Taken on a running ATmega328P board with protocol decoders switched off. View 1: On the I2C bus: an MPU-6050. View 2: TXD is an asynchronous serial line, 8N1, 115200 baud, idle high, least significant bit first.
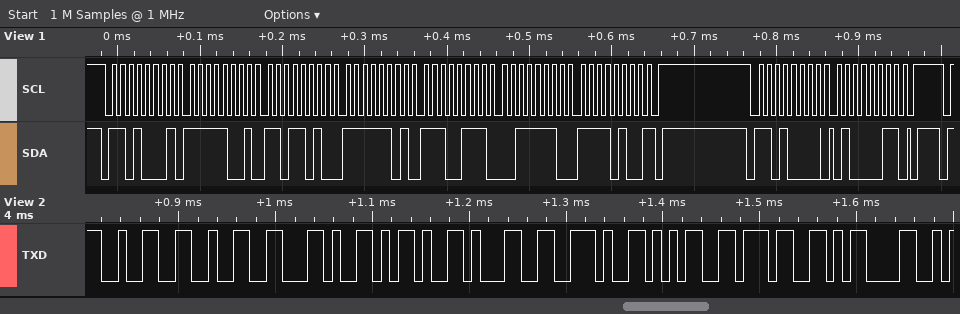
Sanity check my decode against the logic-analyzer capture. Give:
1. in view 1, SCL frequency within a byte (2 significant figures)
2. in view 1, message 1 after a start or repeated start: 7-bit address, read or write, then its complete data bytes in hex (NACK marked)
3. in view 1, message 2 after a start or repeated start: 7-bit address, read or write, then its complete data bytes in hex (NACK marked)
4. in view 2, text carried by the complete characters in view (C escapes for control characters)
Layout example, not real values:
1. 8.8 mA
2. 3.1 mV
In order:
1. 100 kHz
2. 0x68 read: F9 DA FD E7 3E F4 NACK
3. 0x68 write: 43
4. "22,-1.57\r"
